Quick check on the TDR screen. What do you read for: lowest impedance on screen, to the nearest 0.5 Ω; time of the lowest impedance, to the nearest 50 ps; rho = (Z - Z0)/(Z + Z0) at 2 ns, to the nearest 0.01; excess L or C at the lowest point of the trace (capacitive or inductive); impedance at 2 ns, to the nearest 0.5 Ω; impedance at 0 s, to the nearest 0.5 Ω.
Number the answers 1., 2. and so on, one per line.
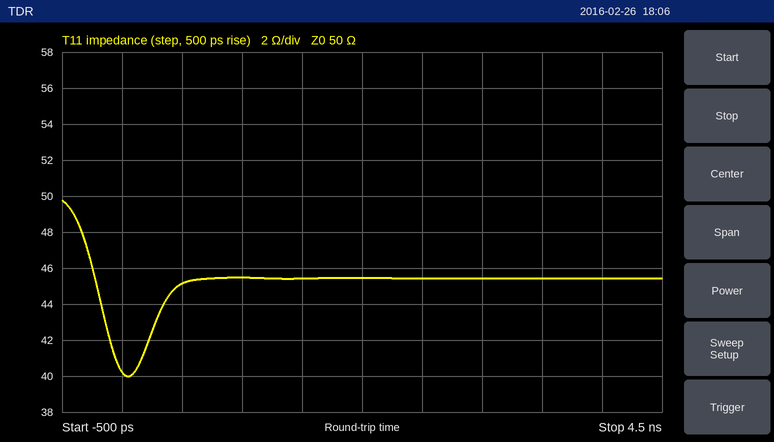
1. 40.0 Ω
2. 50 ps
3. -0.05
4. capacitive
5. 45.5 Ω
6. 40.0 Ω
